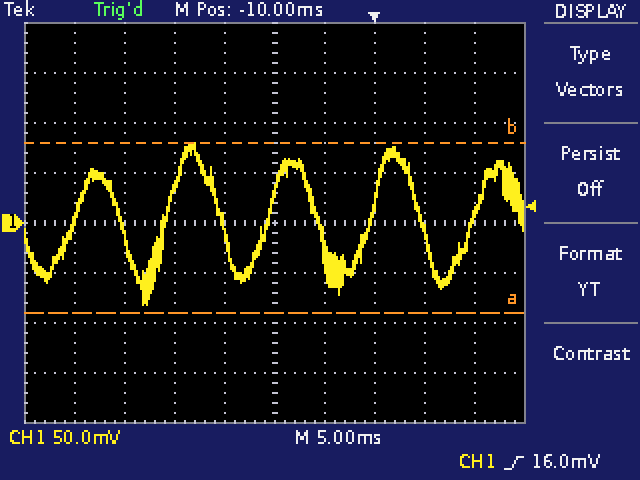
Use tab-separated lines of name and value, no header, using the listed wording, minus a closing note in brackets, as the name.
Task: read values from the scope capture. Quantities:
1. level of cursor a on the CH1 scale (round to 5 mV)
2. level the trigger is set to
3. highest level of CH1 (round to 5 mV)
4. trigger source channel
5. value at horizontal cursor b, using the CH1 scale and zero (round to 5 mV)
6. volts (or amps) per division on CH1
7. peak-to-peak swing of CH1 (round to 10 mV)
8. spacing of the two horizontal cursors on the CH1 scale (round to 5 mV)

level of cursor a on the CH1 scale	-90 mV
level the trigger is set to	16.0 mV
highest level of CH1	80 mV
trigger source channel	CH1
value at horizontal cursor b, using the CH1 scale and zero	80 mV
volts (or amps) per division on CH1	50 mV
peak-to-peak swing of CH1	160 mV
spacing of the two horizontal cursors on the CH1 scale	170 mV
